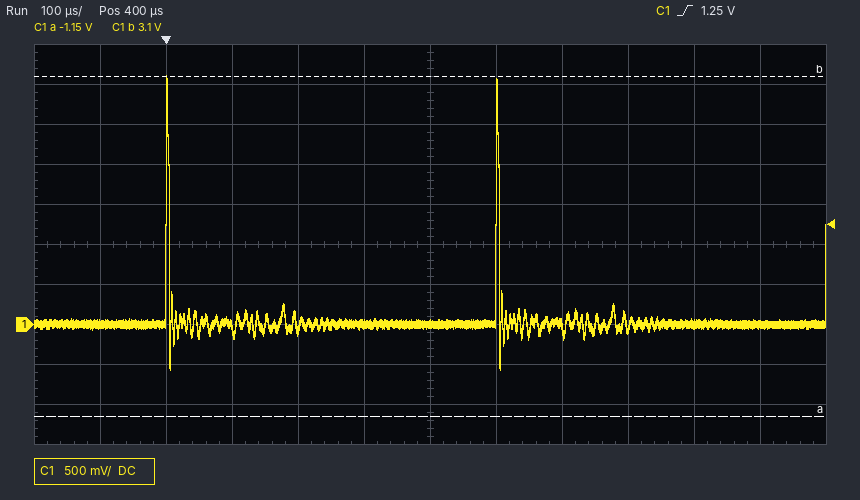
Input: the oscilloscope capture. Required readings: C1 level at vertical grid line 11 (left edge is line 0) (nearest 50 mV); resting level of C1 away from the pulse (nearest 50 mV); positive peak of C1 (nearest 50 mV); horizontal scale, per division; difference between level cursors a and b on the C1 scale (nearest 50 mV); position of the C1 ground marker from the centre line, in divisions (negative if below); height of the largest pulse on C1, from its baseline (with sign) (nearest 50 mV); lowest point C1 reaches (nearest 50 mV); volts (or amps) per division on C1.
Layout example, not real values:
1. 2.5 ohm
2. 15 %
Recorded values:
1. 0 mV
2. 0 mV
3. 3.10 V
4. 100 µs
5. 4.25 V
6. -2.0 div
7. +3.10 V
8. -550 mV
9. 500 mV
